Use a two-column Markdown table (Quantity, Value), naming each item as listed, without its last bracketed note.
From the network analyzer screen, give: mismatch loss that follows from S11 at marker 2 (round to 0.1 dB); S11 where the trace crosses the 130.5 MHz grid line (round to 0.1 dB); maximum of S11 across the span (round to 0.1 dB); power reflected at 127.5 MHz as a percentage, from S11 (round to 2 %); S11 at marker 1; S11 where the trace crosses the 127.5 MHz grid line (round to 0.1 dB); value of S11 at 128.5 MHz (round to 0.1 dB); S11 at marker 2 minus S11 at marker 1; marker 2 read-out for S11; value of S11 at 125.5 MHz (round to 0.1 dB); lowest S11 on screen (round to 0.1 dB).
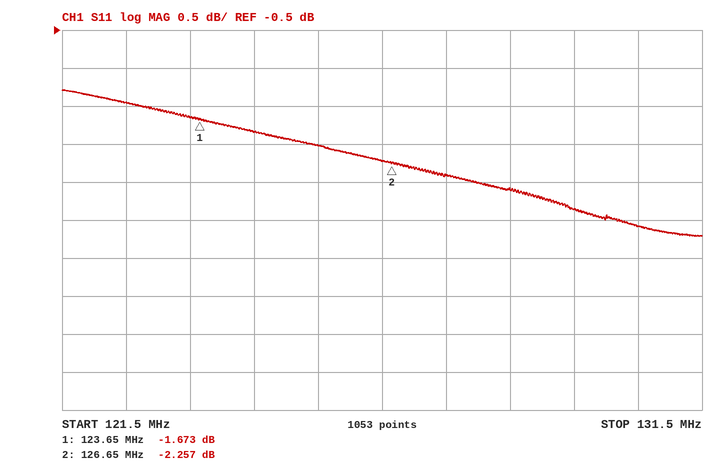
| Quantity | Value |
|---|---|
| mismatch loss that follows from S11 at marker 2 | 3.9 dB |
| S11 where the trace crosses the 130.5 MHz grid line | -3.1 dB |
| maximum of S11 across the span | -1.3 dB |
| power reflected at 127.5 MHz as a percentage, from S11 | 58 % |
| S11 at marker 1 | -1.673 dB |
| S11 where the trace crosses the 127.5 MHz grid line | -2.4 dB |
| value of S11 at 128.5 MHz | -2.6 dB |
| S11 at marker 2 minus S11 at marker 1 | -0.584 dB |
| marker 2 read-out for S11 | -2.257 dB |
| value of S11 at 125.5 MHz | -2.0 dB |
| lowest S11 on screen | -3.2 dB |
